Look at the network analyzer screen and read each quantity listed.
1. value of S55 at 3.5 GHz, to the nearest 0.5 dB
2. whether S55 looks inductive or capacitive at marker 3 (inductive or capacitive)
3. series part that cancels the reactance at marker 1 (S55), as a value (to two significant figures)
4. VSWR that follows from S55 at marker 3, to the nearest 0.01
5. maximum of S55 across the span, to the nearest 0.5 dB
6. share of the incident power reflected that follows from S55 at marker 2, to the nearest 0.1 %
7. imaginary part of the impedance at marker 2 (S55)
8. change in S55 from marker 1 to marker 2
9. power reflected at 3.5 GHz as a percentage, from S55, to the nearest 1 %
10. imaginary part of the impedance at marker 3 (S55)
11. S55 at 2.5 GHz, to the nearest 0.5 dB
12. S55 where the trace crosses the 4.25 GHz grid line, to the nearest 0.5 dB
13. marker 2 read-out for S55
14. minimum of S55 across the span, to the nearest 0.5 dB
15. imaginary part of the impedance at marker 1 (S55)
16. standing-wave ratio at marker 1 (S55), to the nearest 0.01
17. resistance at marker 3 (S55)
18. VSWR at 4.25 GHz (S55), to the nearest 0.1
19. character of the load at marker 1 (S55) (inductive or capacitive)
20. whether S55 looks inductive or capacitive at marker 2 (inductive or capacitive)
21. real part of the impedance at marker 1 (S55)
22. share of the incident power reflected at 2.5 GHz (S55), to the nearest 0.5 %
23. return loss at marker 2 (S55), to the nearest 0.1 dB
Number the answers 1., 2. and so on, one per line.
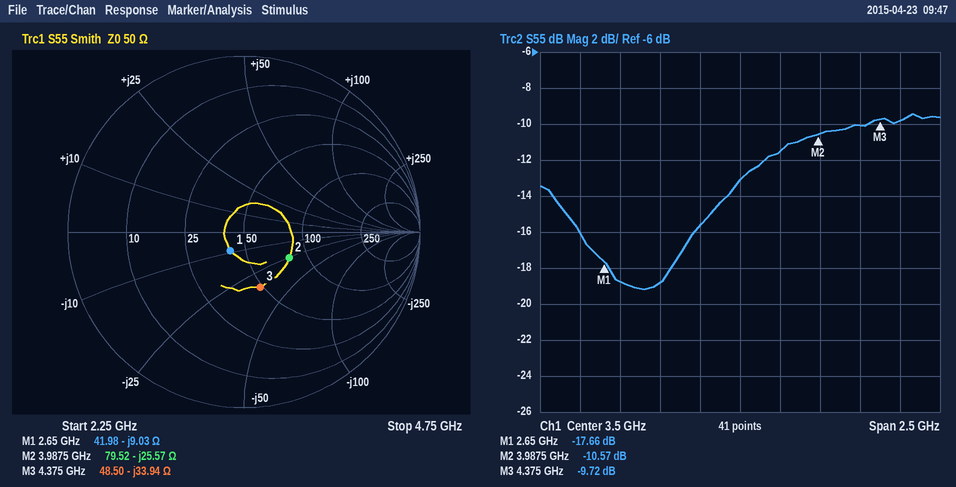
1. -13.0 dB
2. capacitive
3. 540 pH
4. 1.97
5. -9.5 dB
6. 8.8 %
7. -25.57 Ω
8. 7.09 dB
9. 5 %
10. -33.94 Ω
11. -16.0 dB
12. -10.0 dB
13. -10.57 dB
14. -19.0 dB
15. -9.03 Ω
16. 1.30
17. 48.50 Ω
18. 1.9
19. capacitive
20. capacitive
21. 41.98 Ω
22. 2.5 %
23. 10.6 dB
